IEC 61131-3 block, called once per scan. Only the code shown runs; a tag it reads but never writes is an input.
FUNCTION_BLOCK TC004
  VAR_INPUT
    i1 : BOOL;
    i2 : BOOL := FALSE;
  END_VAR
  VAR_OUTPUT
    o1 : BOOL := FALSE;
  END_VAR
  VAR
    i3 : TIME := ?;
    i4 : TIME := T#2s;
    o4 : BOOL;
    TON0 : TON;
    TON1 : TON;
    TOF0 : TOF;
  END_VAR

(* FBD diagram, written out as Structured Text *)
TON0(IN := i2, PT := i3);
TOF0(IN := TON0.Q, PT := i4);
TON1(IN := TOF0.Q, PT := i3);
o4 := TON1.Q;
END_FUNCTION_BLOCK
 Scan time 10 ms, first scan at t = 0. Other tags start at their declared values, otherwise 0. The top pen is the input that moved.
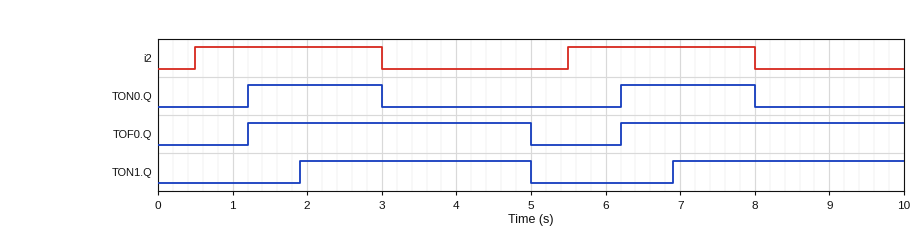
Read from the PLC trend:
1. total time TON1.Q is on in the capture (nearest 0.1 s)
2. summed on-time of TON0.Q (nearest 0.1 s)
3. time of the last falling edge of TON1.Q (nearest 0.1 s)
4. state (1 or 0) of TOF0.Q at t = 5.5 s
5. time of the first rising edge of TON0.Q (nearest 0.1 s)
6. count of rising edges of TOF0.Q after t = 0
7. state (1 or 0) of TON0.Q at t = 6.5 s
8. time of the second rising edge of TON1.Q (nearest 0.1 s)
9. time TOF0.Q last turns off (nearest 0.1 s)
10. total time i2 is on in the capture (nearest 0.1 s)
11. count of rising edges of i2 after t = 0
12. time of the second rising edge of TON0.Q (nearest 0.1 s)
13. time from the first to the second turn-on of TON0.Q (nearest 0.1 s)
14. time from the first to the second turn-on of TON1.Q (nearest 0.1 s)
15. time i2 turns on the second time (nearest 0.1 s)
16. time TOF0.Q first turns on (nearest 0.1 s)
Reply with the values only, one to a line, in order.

6.2 s
3.6 s
5.0 s
0
1.2 s
2
1
6.9 s
5.0 s
5.0 s
2
6.2 s
5.0 s
5.0 s
5.5 s
1.2 s
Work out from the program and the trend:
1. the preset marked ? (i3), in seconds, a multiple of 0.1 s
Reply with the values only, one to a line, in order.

0.7 s
